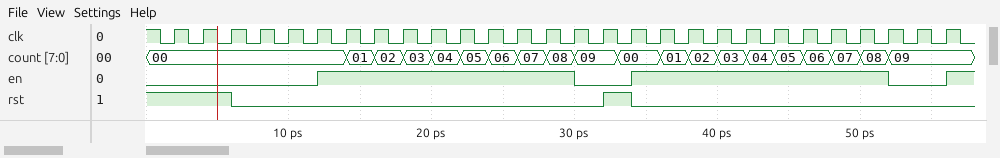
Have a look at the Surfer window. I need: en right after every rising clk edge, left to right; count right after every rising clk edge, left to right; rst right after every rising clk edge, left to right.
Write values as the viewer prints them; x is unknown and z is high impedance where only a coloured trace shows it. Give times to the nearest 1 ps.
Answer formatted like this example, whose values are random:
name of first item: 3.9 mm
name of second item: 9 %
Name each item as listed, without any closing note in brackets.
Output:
en right after every rising clk edge, left to right: 0 0 0 0 0 1 1 1 1 1 1 1 1 1 0 0 1 1 1 1 1 1 1 1 1 0 0 1
count right after every rising clk edge, left to right: 00, 00, 00, 00, 00, 00, 01, 02, 03, 04, 05, 06, 07, 08, 09, 09, 00, 01, 02, 03, 04, 05, 06, 07, 08, 09, 09, 09
rst right after every rising clk edge, left to right: 1 1 0 0 0 0 0 0 0 0 0 0 0 0 0 1 0 0 0 0 0 0 0 0 0 0 0 0
